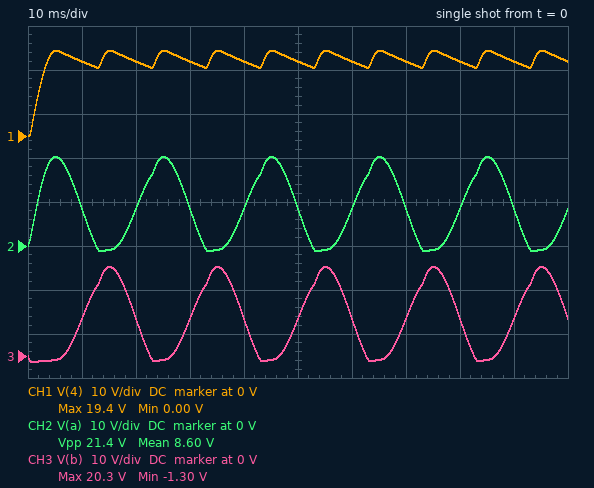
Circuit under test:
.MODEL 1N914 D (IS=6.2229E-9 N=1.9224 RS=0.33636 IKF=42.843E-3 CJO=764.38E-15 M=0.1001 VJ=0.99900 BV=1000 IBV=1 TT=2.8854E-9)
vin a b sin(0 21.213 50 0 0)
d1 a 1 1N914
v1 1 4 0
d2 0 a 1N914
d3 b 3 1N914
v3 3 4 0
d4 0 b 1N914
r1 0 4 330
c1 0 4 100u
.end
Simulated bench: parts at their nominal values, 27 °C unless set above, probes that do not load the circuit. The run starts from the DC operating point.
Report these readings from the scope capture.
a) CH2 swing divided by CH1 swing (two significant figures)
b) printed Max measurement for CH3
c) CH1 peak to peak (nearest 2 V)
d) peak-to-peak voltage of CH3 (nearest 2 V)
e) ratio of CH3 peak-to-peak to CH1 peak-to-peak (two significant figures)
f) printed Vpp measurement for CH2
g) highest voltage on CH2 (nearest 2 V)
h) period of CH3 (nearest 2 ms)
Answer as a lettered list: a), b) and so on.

a) 1.1
b) 20.3 V
c) 20 V
d) 22 V
e) 1.1
f) 21.4 V
g) 20 V
h) 20 ms
